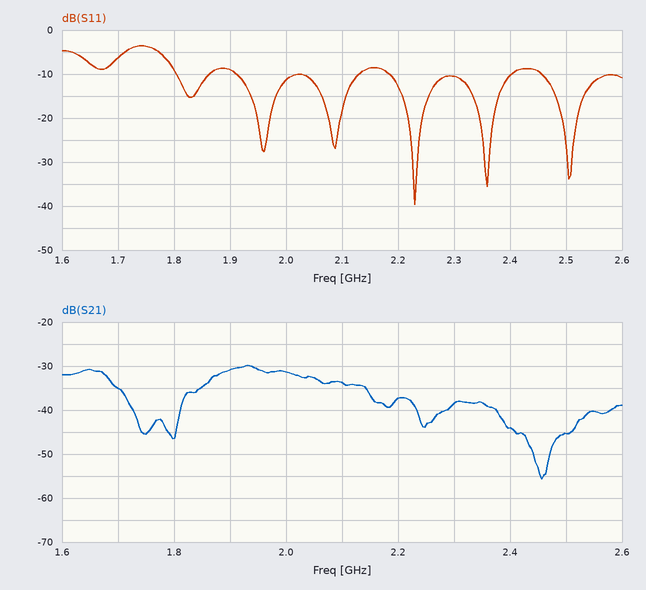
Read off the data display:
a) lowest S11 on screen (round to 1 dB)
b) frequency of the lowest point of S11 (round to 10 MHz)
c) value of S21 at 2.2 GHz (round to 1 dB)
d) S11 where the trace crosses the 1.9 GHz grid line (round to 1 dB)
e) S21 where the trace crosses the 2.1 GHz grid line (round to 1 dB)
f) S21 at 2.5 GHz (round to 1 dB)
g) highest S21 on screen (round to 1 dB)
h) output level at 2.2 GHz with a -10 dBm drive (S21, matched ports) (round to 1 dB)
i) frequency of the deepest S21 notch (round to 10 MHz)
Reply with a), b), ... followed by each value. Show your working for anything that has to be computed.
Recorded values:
a) -40 dB
b) 2.23 GHz
c) -37 dB
d) -9 dB
e) -34 dB
f) -45 dB
g) -30 dB
h) -10 dBm + (-37 dB) = -47 dBm
i) 2.46 GHz
